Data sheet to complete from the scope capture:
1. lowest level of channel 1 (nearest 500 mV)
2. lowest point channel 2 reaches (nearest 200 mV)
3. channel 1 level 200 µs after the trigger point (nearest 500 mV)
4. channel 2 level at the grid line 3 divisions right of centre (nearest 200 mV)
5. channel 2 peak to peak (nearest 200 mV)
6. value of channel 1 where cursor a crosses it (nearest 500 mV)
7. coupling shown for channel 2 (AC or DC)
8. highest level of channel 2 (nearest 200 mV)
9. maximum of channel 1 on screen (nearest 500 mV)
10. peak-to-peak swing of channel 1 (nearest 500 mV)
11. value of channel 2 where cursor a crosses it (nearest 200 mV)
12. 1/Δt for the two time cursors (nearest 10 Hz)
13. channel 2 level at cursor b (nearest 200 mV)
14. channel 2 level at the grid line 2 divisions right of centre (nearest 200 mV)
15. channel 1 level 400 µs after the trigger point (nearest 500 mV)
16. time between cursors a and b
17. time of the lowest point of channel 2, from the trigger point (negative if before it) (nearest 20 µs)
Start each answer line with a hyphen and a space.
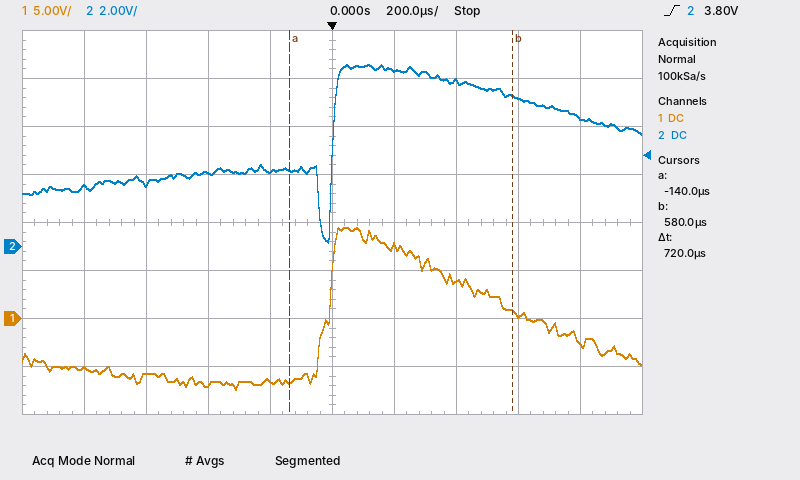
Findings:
- -7.5 V
- 200 mV
- 7.5 V
- 6.2 V
- 7.4 V
- -6.5 V
- DC
- 7.6 V
- 9.5 V
- 17.0 V
- 3.2 V
- 1.39 kHz
- 6.2 V
- 6.8 V
- 4.0 V
- 720 µs
- -20 µs
